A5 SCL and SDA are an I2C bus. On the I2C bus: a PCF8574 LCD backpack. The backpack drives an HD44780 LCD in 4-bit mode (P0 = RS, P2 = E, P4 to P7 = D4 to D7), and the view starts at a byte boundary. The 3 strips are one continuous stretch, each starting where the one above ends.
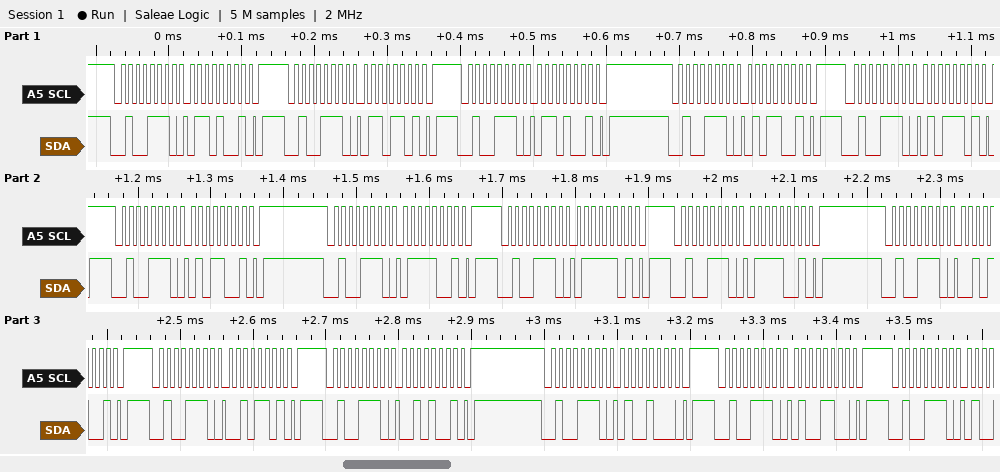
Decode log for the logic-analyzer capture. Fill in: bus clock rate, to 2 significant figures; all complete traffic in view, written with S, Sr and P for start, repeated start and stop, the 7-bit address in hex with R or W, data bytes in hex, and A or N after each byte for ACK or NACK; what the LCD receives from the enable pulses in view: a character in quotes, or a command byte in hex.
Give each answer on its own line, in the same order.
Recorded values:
100 kHz
S 27W A 69 A P S 27W A 6D A P S 27W A 69 A P S 27W A 59 A P S 27W A 5D A P S 27W A 59 A P S 27W A 79 A P S 27W A 7D A P S 27W A 79 A P S 27W A 29 A P S 27W A 2D A P S 27W A 29 A P S 27W A 48 A P S 27W A 4C A P S 27W A
'e' 'r'
